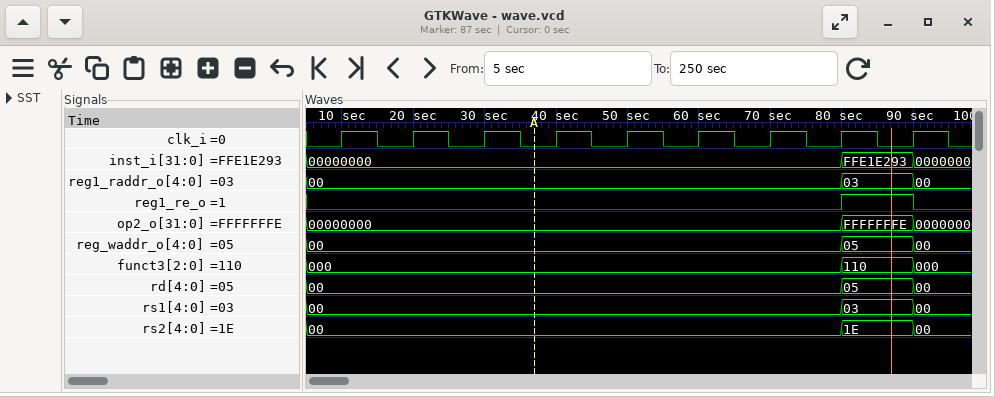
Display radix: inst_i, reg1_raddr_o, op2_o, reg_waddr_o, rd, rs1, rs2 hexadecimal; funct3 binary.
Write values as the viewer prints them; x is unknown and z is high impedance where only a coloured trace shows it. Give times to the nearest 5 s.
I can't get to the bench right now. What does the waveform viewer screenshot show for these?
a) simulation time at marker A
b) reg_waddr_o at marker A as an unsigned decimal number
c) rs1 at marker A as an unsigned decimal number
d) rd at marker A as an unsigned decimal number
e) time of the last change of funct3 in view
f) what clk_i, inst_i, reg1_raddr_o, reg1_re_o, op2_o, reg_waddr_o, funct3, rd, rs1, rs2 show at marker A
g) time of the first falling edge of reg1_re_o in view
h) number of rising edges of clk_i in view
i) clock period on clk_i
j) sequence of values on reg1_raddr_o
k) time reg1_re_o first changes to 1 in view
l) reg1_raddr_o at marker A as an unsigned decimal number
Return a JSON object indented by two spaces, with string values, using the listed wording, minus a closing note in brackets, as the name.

{
  "simulation time at marker A": "35 s",
  "reg_waddr_o at marker A as an unsigned decimal number": "0",
  "rs1 at marker A as an unsigned decimal number": "0",
  "rd at marker A as an unsigned decimal number": "0",
  "time of the last change of funct3 in view": "90 s",
  "what clk_i, inst_i, reg1_raddr_o, reg1_re_o, op2_o, reg_waddr_o, funct3, rd, rs1, rs2 show at marker A": "clk_i=0, inst_i=00000000, reg1_raddr_o=00, reg1_re_o=0, op2_o=00000000, reg_waddr_o=00, funct3=000, rd=00, rs1=00, rs2=00",
  "time of the first falling edge of reg1_re_o in view": "90 s",
  "number of rising edges of clk_i in view": "9",
  "clock period on clk_i": "10 s",
  "sequence of values on reg1_raddr_o": "00, 03, 00",
  "time reg1_re_o first changes to 1 in view": "80 s",
  "reg1_raddr_o at marker A as an unsigned decimal number": "0"
}
